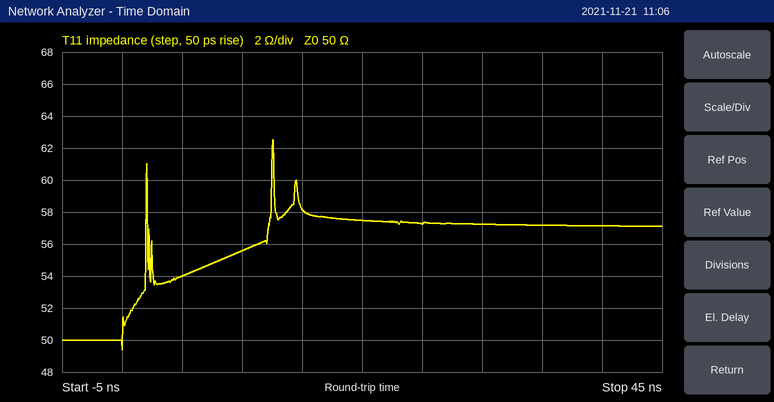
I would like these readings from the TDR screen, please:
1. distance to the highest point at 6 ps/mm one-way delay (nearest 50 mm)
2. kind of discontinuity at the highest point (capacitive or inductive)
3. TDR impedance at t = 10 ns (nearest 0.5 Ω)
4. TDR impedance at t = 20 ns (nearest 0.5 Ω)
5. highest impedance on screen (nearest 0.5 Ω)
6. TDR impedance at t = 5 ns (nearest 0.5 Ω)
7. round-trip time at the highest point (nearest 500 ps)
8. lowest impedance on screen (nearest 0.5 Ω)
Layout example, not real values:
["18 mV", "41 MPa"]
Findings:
["1.05 m", "inductive", "55.5 Ω", "57.5 Ω", "62.5 Ω", "54.0 Ω", "12.5 ns", "49.5 Ω"]
